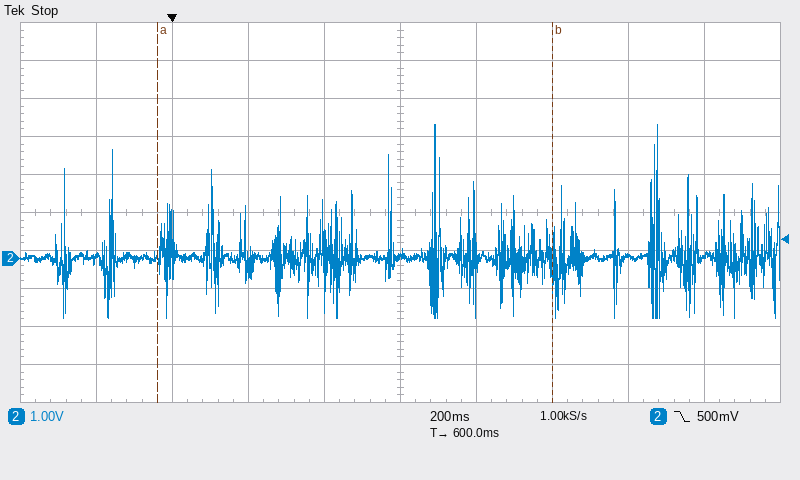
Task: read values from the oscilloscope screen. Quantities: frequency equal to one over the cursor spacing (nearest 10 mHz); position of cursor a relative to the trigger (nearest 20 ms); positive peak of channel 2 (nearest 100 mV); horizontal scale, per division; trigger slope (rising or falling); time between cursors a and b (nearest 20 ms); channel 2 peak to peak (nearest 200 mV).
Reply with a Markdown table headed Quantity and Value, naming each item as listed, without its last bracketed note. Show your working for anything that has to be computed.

| Quantity | Value |
|---|---|
| frequency equal to one over the cursor spacing | 1 / 1.04 s ≈ 960 mHz |
| position of cursor a relative to the trigger | -40 ms |
| positive peak of channel 2 | 3.5 V |
| horizontal scale, per division | 200 ms |
| trigger slope | falling |
| time between cursors a and b | 1.04 s |
| channel 2 peak to peak | 5.0 V |
